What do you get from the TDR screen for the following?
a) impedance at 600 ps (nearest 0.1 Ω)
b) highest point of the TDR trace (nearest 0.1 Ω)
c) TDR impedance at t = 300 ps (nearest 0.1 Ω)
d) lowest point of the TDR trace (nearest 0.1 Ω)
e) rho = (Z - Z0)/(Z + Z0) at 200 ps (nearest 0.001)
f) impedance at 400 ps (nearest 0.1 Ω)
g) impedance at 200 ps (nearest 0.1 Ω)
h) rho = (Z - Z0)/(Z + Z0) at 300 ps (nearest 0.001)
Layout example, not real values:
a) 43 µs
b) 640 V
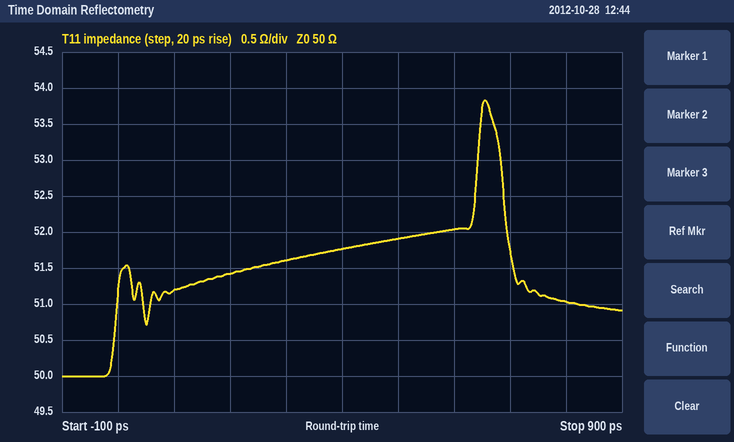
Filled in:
a) 52.0 Ω
b) 53.8 Ω
c) 51.6 Ω
d) 50.0 Ω
e) +0.014
f) 51.8 Ω
g) 51.4 Ω
h) +0.016
